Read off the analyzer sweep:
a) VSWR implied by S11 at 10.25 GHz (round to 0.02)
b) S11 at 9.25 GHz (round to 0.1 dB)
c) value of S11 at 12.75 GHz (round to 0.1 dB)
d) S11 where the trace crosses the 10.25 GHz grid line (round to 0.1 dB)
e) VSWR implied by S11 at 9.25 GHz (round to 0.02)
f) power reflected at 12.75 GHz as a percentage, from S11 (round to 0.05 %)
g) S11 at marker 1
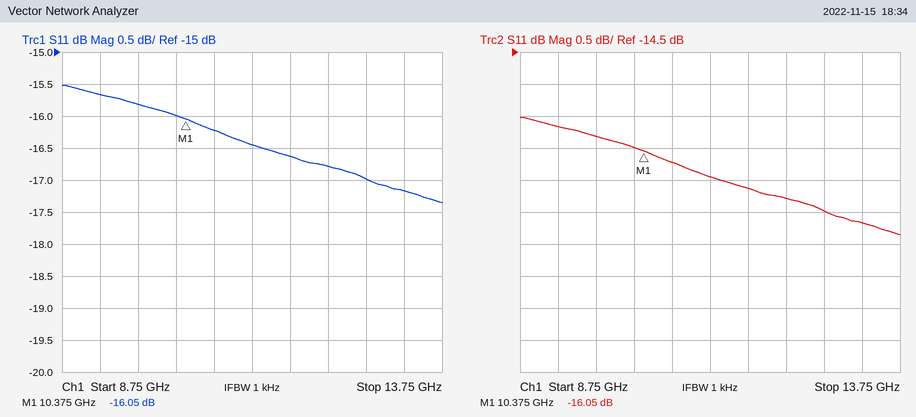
1.38
-15.7 dB
-17.0 dB
-16.0 dB
1.40
2.00 %
-16.05 dB
